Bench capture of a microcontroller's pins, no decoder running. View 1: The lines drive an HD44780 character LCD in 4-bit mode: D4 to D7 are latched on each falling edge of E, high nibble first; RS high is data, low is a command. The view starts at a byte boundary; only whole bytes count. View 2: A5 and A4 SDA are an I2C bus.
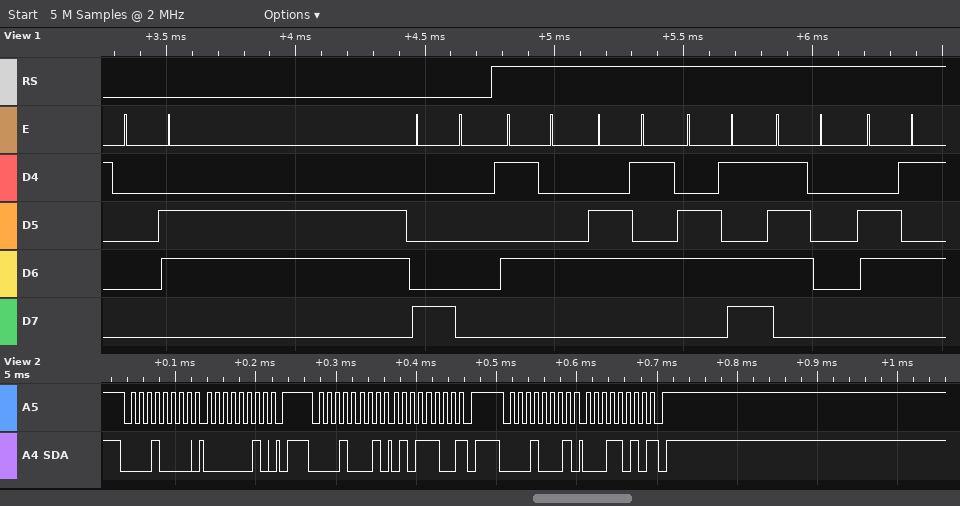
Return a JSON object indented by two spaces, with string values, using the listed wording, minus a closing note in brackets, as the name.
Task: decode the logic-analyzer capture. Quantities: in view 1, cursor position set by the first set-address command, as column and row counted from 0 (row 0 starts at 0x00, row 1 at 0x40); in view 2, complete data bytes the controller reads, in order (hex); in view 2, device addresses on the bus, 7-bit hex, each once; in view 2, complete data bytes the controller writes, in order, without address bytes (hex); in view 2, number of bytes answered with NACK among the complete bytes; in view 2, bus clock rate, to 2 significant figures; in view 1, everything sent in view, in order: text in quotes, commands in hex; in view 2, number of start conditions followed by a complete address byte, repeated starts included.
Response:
{
  "in view 1, cursor position set by the first set-address command, as column and row counted from 0": "column 0, row 0",
  "in view 2, complete data bytes the controller reads, in order": "5C 1A",
  "in view 2, device addresses on the bus, 7-bit hex, each once": "0x08",
  "in view 2, complete data bytes the controller writes, in order, without address bytes": "02",
  "in view 2, number of bytes answered with NACK among the complete bytes": "2",
  "in view 2, bus clock rate, to 2 significant figures": "100 kHz",
  "in view 1, everything sent in view, in order: text in quotes, commands in hex": "0x06 0x80 \"Tempe\"",
  "in view 2, number of start conditions followed by a complete address byte, repeated starts included": "3"
}
